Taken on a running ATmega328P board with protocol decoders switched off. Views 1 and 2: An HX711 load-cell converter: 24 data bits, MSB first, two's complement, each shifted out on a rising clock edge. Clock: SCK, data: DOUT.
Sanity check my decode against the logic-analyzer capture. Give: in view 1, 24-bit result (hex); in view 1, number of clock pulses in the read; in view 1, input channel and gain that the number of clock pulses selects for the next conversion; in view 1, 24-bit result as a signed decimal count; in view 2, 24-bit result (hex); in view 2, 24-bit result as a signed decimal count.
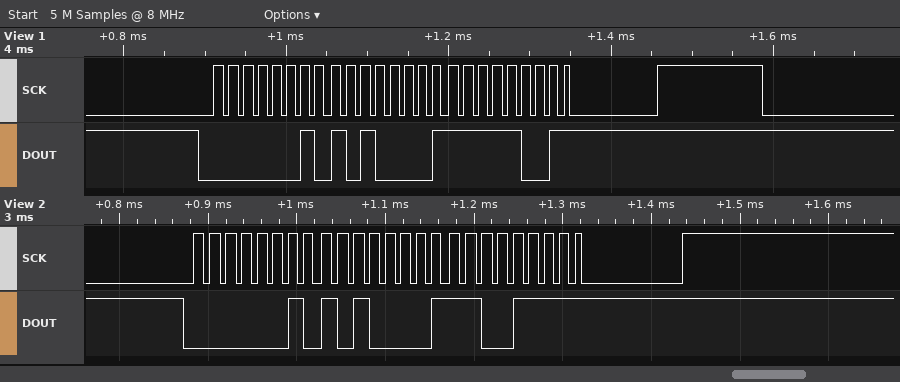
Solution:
0x02A1F9
26
channel B, gain 32
172537
0x02A1CF
172495
